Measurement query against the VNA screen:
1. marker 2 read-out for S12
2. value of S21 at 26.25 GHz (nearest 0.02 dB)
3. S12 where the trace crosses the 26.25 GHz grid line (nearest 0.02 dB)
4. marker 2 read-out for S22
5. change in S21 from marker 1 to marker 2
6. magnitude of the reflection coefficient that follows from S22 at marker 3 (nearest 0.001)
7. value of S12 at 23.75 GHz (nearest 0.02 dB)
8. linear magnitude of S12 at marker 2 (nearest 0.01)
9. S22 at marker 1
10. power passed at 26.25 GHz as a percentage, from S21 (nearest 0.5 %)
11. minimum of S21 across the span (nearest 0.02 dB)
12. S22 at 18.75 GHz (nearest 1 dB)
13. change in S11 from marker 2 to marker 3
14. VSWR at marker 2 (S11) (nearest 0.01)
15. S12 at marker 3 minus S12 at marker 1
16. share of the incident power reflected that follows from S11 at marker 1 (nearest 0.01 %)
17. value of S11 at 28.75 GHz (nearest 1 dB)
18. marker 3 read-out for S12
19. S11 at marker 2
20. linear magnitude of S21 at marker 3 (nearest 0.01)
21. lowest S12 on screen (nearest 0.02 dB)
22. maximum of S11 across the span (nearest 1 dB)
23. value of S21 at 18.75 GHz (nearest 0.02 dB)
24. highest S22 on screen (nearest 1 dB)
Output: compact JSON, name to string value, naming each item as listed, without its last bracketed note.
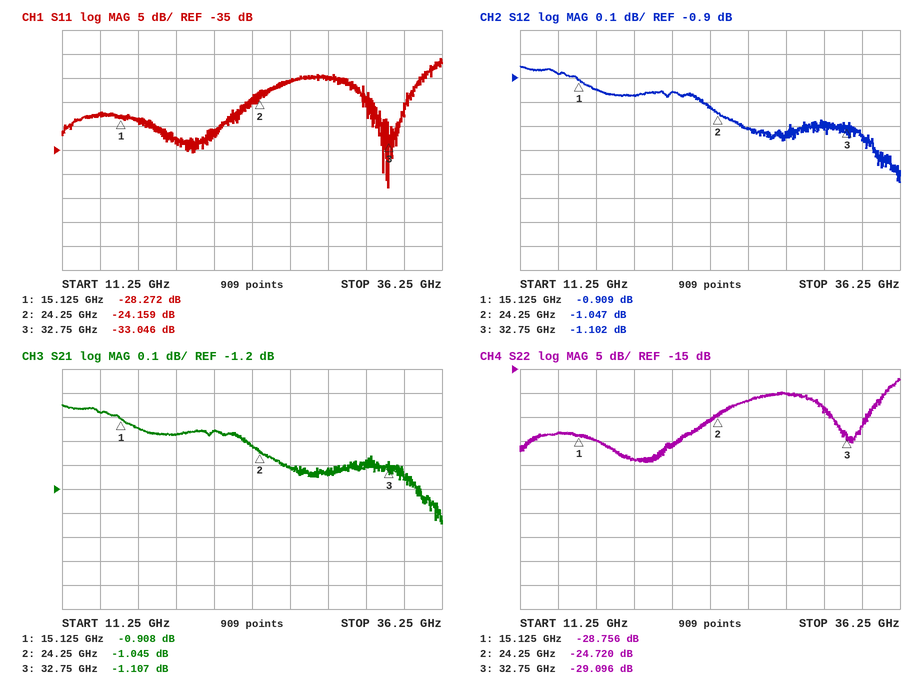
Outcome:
{"marker 2 read-out for S12": "-1.047 dB", "value of S21 at 26.25 GHz": "-1.12 dB", "S12 where the trace crosses the 26.25 GHz grid line": "-1.10 dB", "marker 2 read-out for S22": "-24.720 dB", "change in S21 from marker 1 to marker 2": "-0.137 dB", "magnitude of the reflection coefficient that follows from S22 at marker 3": "0.035", "value of S12 at 23.75 GHz": "-1.02 dB", "linear magnitude of S12 at marker 2": "0.89", "S22 at marker 1": "-28.756 dB", "power passed at 26.25 GHz as a percentage, from S21": "77.5 %", "minimum of S21 across the span": "-1.34 dB", "S22 at 18.75 GHz": "-34 dB", "change in S11 from marker 2 to marker 3": "-8.887 dB", "VSWR at marker 2 (S11)": "1.13", "S12 at marker 3 minus S12 at marker 1": "-0.193 dB", "share of the incident power reflected that follows from S11 at marker 1": "0.15 %", "value of S11 at 28.75 GHz": "-20 dB", "marker 3 read-out for S12": "-1.102 dB", "S11 at marker 2": "-24.159 dB", "linear magnitude of S21 at marker 3": "0.88", "lowest S12 on screen": "-1.34 dB", "maximum of S11 across the span": "-16 dB", "value of S21 at 18.75 GHz": "-0.98 dB", "highest S22 on screen": "-17 dB"}
